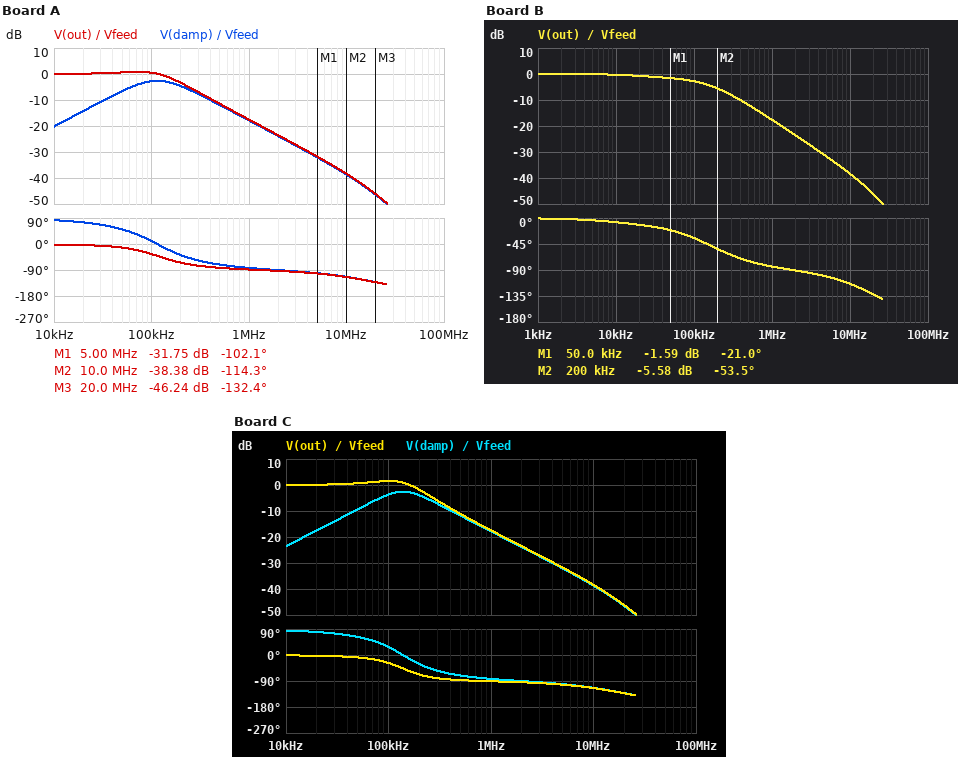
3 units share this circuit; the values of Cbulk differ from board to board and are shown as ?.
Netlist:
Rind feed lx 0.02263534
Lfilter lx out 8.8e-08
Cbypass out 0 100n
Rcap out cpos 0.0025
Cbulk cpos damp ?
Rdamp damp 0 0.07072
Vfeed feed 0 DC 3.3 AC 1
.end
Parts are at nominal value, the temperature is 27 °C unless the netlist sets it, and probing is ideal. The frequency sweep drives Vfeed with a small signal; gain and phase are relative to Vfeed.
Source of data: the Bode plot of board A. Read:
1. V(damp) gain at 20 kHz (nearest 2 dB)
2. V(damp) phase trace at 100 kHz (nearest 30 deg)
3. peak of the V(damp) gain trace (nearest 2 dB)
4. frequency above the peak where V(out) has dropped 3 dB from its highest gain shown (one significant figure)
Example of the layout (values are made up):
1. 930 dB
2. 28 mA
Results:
1. -14 dB
2. 0 deg
3. -2 dB
4. 200 kHz
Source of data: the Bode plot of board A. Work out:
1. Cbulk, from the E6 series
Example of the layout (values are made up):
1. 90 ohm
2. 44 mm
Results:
1. 22 µF
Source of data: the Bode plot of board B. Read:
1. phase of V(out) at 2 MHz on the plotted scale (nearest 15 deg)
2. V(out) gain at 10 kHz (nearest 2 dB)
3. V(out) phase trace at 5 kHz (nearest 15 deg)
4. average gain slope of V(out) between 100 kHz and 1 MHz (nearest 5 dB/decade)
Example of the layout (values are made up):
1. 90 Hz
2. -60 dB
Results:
1. -90 deg
2. 0 dB
3. 0 deg
4. -15 dB/decade
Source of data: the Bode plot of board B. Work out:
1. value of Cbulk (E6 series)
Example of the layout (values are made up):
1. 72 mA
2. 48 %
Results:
1. 100 µF
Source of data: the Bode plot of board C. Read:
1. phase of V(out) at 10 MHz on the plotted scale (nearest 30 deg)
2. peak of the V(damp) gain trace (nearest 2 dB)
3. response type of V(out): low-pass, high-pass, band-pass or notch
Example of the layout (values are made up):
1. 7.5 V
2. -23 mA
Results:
1. -120 deg
2. -2 dB
3. low-pass
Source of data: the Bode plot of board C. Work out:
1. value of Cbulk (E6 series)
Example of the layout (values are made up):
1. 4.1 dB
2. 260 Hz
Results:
1. 15 µF
